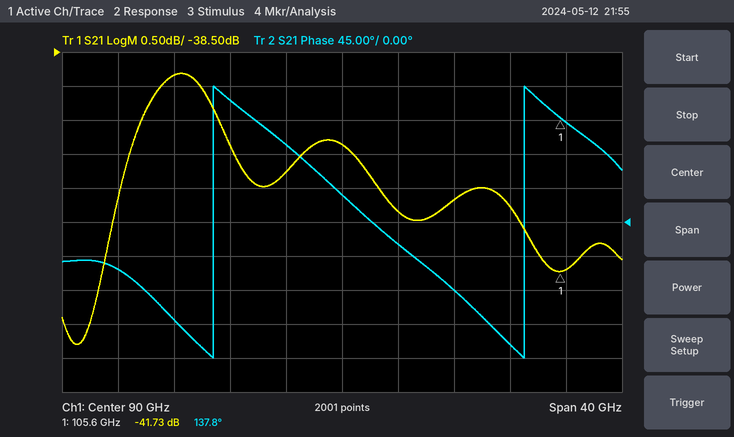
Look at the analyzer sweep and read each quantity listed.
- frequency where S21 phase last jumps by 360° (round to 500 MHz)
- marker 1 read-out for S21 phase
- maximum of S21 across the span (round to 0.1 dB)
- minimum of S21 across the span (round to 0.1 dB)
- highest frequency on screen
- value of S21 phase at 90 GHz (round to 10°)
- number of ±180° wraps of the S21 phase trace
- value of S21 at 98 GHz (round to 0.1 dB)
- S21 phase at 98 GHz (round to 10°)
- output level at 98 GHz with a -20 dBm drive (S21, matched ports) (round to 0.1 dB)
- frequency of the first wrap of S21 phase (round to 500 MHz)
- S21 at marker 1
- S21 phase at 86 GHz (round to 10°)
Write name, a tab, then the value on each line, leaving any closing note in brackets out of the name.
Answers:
frequency where S21 phase last jumps by 360°	103.0 GHz
marker 1 read-out for S21 phase	137.8°
maximum of S21 across the span	-38.8 dB
minimum of S21 across the span	-42.8 dB
highest frequency on screen	110 GHz
value of S21 phase at 90 GHz	40°
number of ±180° wraps of the S21 phase trace	2
value of S21 at 98 GHz	-40.7 dB
S21 phase at 98 GHz	-90°
output level at 98 GHz with a -20 dBm drive (S21, matched ports)	-60.7 dBm
frequency of the first wrap of S21 phase	81.0 GHz
S21 at marker 1	-41.73 dB
S21 phase at 86 GHz	100°
